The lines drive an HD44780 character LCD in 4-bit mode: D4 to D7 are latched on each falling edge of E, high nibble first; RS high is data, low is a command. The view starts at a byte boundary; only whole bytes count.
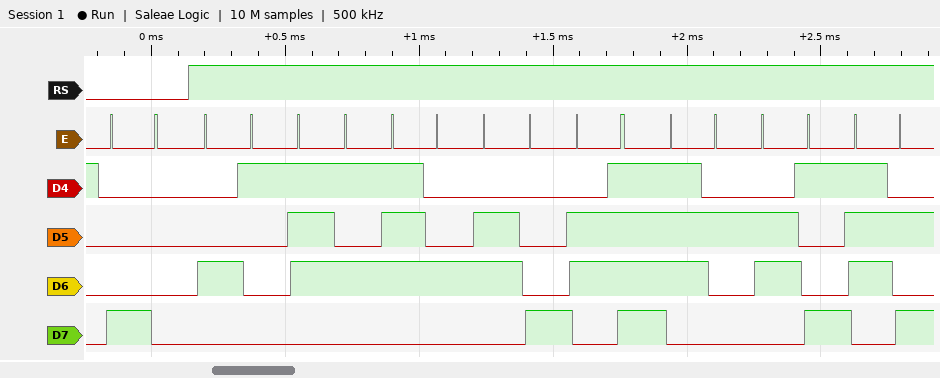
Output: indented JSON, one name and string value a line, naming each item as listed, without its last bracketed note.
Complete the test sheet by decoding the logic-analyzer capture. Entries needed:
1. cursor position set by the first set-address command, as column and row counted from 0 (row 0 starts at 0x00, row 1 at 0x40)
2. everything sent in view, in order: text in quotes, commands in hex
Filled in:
{
  "cursor position set by the first set-address command, as column and row counted from 0": "column 0, row 0",
  "everything sent in view, in order: text in quotes, commands in hex": "0x80 \"Authoriz\""
}
